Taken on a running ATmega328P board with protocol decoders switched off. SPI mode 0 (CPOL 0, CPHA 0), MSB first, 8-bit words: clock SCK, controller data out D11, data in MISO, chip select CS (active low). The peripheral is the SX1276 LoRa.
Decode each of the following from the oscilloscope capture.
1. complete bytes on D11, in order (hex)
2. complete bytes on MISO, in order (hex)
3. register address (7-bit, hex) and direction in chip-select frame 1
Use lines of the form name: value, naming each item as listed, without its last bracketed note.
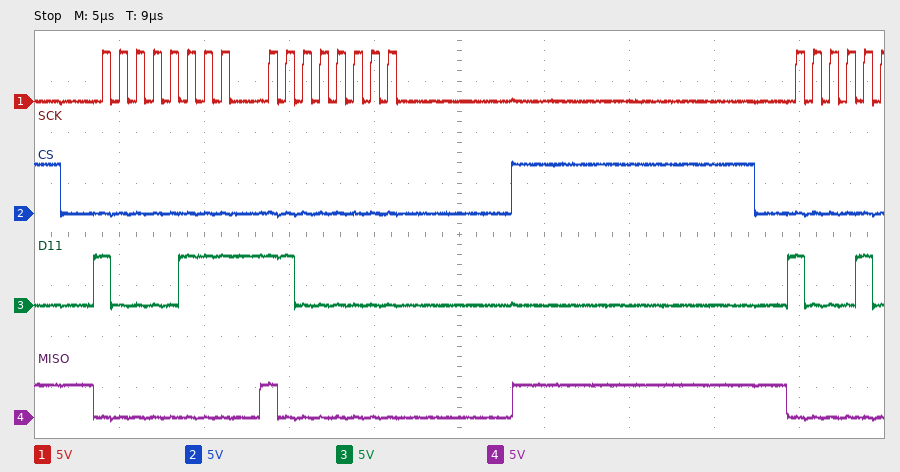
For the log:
complete bytes on D11, in order: 0x87 0xC0
complete bytes on MISO, in order: 0x00 0x80
register address (7-bit, hex) and direction in chip-select frame 1: 0x07 write
